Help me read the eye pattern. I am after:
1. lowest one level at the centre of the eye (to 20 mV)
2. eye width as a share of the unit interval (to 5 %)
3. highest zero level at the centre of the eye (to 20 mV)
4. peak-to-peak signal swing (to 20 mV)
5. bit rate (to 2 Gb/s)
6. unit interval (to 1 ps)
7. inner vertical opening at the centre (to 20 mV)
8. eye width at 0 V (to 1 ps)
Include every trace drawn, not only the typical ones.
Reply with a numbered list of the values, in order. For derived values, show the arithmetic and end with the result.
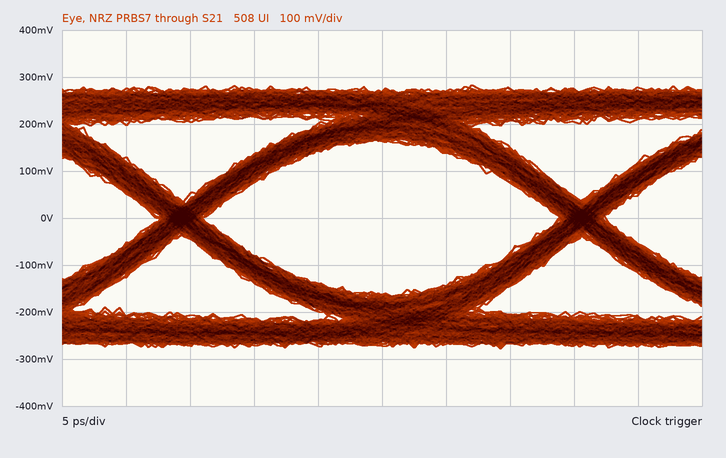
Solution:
1. 160 mV
2. 28 ps / 31 ps ≈ 90 %
3. -160 mV
4. 560 mV
5. 32 Gb/s
6. 31 ps
7. 320 mV
8. 28 ps
